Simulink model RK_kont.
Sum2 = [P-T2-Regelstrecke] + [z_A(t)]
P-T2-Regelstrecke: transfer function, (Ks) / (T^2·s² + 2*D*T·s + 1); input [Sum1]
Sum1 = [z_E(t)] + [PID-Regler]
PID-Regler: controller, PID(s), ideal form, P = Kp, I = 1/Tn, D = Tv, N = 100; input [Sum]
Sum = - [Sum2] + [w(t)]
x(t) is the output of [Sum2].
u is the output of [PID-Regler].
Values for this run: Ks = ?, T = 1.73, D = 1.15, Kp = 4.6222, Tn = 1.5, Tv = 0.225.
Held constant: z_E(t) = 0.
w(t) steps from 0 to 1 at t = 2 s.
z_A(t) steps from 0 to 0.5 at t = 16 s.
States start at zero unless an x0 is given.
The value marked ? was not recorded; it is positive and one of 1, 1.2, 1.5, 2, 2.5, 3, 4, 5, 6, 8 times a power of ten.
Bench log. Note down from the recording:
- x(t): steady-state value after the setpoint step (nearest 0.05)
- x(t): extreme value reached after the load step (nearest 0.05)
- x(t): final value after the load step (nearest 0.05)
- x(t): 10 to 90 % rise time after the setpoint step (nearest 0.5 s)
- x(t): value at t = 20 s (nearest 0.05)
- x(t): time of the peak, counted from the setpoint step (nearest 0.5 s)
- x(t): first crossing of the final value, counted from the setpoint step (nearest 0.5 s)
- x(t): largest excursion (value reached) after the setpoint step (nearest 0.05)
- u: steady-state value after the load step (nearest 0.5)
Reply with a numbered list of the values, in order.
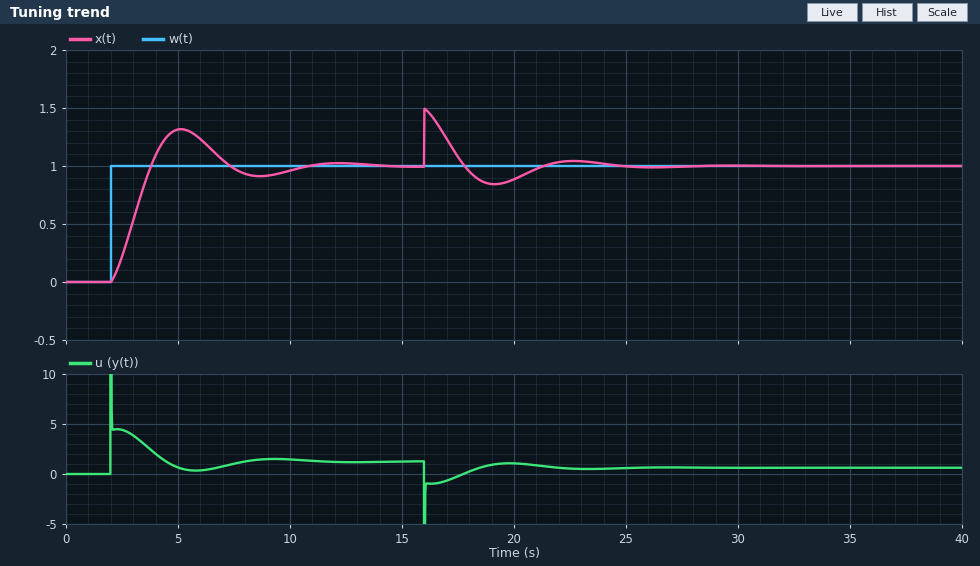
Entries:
1. 1.00
2. 1.50
3. 1.00
4. 1.5 s
5. 0.90
6. 3.0 s
7. 2.0 s
8. 1.30
9. 0.5
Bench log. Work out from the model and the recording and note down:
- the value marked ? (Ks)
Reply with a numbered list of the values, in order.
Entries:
1. 0.8
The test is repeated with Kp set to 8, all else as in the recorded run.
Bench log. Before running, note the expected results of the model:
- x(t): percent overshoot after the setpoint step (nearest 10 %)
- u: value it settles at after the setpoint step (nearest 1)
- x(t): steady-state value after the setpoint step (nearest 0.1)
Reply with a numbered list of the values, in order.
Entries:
1. 30 %
2. 1
3. 1.0
